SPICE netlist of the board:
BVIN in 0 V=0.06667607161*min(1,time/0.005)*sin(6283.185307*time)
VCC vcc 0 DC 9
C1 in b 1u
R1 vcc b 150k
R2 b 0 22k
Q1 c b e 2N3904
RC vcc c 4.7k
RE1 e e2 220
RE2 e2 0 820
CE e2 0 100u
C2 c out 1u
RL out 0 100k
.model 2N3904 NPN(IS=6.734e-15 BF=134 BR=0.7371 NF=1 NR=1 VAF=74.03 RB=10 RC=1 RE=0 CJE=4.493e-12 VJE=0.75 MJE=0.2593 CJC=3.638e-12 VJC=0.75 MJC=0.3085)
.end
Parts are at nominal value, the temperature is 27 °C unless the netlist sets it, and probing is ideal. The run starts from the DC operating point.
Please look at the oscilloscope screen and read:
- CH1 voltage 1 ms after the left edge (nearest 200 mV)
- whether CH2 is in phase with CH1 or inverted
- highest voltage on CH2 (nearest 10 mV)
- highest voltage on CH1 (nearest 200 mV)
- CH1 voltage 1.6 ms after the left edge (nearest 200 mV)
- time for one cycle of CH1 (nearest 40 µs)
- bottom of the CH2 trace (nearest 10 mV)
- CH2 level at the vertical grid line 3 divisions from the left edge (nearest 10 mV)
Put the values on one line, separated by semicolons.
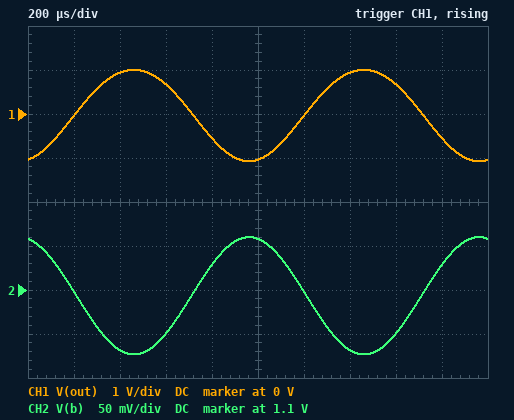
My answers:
-1.0 V; inverted; 1.16 V; 1.0 V; 600 mV; 1.00 ms; 1.03 V; 1.05 V
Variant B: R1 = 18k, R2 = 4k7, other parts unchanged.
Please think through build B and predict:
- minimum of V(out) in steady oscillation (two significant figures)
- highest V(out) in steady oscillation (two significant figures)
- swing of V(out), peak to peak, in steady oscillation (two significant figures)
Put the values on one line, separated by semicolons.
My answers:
-1.2 V; 1.2 V; 2.4 V
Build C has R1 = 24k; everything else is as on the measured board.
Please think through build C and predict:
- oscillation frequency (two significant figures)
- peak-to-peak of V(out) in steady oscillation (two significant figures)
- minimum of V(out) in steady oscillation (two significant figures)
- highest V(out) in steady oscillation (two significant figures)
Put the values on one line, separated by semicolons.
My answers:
1.0 kHz; 470 mV; -52 mV; 420 mV
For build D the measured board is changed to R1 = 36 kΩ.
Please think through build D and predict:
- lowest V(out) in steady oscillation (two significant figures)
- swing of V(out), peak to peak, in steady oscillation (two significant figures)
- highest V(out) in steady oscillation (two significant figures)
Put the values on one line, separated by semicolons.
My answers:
-200 mV; 1.3 V; 1.1 V
